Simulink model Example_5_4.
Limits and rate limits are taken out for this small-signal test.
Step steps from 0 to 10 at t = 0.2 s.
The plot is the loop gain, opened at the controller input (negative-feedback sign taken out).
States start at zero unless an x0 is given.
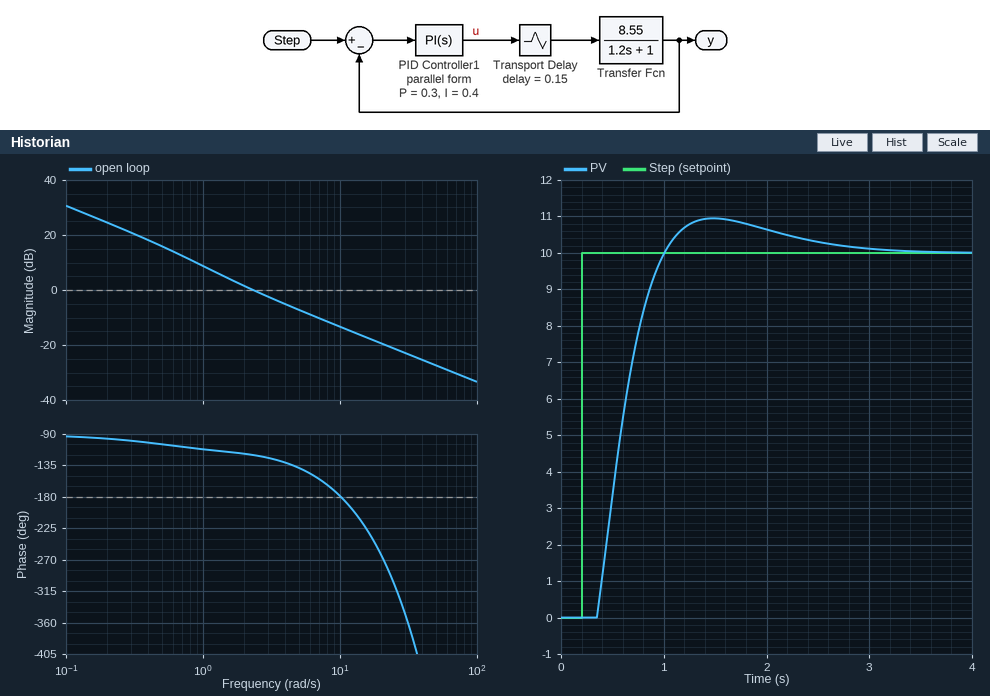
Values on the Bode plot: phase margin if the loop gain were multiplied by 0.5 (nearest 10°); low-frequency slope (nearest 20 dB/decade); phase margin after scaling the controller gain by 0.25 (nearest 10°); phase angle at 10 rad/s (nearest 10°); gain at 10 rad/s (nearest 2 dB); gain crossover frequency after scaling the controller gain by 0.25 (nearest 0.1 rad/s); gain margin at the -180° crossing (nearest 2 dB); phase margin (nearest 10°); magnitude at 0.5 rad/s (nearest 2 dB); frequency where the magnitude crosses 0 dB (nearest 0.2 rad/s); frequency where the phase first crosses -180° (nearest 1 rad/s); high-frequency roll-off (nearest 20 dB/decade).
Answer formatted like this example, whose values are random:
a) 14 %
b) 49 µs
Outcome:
a) 70°
b) -20 dB/decade
c) 70°
d) -180°
e) -14 dB
f) 0.7 rad/s
g) 14 dB
h) 60°
i) 16 dB
j) 2.4 rad/s
k) 10 rad/s
l) -20 dB/decade
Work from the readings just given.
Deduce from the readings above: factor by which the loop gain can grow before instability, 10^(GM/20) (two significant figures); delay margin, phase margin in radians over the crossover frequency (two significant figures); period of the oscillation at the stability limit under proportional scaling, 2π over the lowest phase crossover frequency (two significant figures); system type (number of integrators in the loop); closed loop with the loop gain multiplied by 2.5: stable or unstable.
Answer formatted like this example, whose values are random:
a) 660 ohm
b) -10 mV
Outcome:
a) 5.0
b) 0.44 s
c) 0.63 s
d) 1
e) stable
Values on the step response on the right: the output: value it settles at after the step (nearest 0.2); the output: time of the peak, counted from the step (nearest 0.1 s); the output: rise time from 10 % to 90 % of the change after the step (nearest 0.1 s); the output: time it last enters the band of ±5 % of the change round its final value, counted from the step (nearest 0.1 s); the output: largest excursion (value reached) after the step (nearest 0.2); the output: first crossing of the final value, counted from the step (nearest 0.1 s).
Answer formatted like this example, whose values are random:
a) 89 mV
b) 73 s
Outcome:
a) 10.0
b) 1.3 s
c) 0.5 s
d) 2.0 s
e) 11.0
f) 0.8 s
